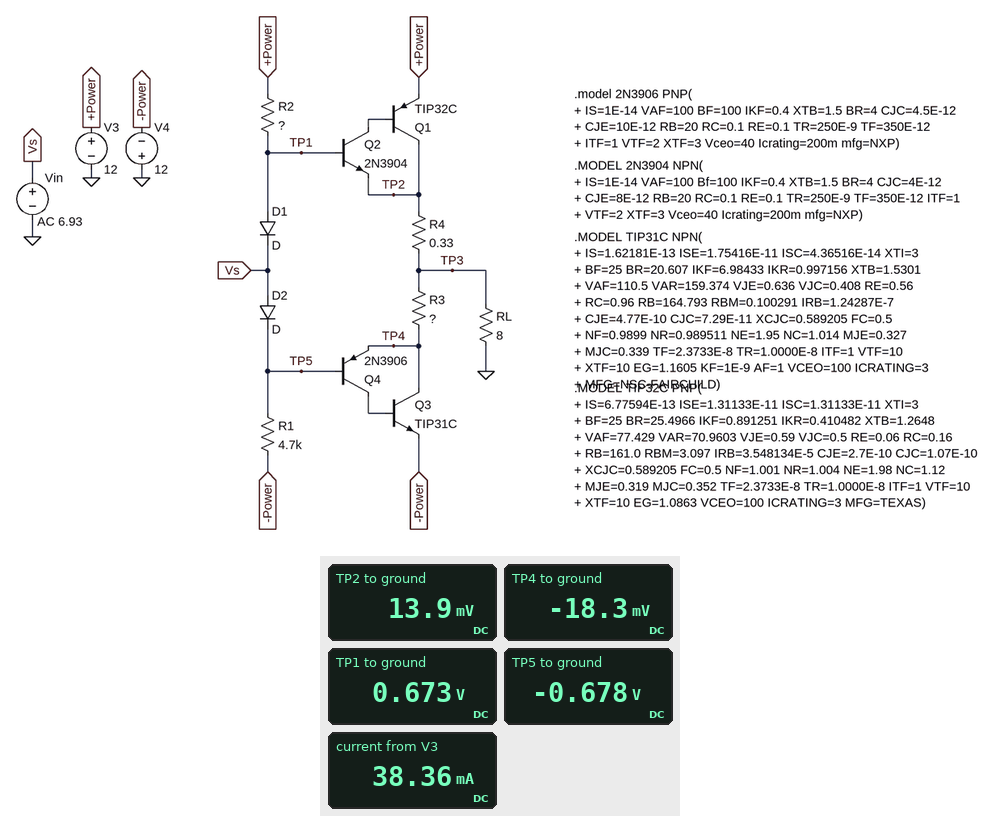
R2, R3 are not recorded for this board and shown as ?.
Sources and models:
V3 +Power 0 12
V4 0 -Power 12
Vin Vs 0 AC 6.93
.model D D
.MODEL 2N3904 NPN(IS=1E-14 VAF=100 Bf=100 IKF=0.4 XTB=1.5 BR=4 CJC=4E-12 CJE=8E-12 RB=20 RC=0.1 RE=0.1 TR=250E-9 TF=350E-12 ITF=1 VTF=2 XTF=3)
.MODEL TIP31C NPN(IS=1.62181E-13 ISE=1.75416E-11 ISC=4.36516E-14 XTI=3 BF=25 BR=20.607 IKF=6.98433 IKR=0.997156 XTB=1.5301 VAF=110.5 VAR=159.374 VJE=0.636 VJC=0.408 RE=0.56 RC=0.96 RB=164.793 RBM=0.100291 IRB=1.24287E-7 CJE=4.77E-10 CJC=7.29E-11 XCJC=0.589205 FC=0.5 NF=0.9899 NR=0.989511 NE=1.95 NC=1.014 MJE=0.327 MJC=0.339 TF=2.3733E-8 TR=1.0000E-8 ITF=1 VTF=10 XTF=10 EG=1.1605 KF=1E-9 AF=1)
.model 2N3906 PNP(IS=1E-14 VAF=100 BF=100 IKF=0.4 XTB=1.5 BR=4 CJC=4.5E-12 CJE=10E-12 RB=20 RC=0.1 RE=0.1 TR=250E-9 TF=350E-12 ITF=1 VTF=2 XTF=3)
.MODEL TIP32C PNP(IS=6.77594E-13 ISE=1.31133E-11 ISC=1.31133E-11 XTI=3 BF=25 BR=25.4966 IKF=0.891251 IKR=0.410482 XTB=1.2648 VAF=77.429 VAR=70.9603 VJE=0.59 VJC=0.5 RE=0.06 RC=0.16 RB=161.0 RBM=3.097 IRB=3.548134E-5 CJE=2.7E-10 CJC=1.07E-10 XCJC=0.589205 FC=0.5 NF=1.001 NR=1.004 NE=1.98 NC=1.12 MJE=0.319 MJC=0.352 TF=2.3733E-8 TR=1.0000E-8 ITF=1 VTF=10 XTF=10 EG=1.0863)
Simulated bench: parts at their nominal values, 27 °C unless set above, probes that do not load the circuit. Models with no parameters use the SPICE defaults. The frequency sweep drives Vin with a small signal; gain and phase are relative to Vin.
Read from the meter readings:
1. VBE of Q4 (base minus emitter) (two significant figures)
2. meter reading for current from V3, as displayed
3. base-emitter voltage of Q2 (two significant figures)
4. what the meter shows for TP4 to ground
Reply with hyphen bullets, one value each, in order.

- -660 mV
- 38.36 mA
- 660 mV
- -18.3 mV
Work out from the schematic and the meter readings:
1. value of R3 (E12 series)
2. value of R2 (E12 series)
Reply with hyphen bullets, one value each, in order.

- 0.56 Ω
- 5.6 kΩ
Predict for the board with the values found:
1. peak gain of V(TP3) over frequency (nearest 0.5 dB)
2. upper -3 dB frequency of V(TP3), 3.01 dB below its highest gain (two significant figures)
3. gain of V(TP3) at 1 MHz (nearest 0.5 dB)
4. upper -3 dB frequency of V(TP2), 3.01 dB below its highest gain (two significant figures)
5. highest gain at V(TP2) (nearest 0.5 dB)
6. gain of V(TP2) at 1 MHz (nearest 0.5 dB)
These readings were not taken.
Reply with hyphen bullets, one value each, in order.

- -0.5 dB
- 4.1 MHz
- -1.0 dB
- 4.1 MHz
- -0.5 dB
- -1.0 dB
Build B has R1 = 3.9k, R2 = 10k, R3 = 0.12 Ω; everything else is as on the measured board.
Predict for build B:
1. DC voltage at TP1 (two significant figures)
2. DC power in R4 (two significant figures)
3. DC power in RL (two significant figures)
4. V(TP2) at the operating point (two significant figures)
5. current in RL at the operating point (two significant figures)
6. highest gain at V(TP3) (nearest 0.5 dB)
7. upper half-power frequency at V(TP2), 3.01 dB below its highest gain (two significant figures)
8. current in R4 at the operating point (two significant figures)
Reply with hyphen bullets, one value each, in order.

- 660 mV
- 490 µW
- 30 µW
- -2.7 mV
- 1.9 mA
- -0.5 dB
- 4.4 MHz
- 38 mA
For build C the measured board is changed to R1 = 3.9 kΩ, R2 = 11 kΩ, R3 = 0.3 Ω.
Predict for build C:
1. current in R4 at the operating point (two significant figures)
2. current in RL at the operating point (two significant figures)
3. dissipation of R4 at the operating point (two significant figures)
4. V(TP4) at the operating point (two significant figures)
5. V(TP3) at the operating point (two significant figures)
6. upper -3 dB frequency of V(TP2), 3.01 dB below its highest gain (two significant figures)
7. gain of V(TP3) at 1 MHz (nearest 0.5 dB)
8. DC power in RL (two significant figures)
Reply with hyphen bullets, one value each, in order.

- 34 mA
- 1.6 mA
- 380 µW
- -24 mV
- -13 mV
- 3.9 MHz
- -1.0 dB
- 21 µW
